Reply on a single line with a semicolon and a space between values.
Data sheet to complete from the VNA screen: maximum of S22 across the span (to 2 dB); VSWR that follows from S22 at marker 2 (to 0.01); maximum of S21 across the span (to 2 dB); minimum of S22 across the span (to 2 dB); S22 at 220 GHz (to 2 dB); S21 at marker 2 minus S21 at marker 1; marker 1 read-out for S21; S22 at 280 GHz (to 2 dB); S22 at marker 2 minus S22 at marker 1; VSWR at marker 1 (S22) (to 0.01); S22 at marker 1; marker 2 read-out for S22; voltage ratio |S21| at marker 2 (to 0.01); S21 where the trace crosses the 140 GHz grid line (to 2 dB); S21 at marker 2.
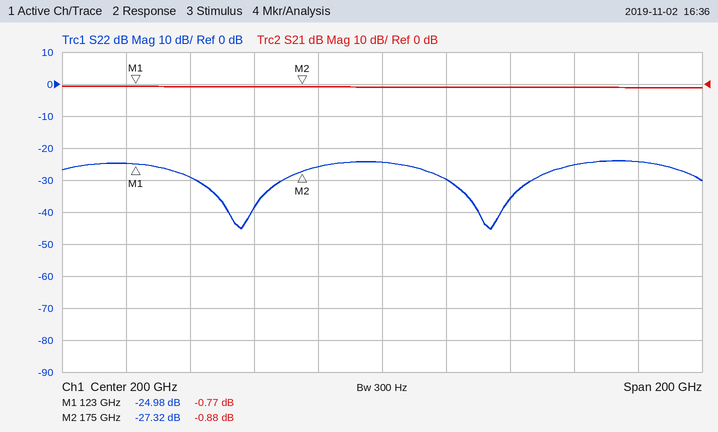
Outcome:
-24 dB; 1.09; 0 dB; -46 dB; -30 dB; -0.11 dB; -0.77 dB; -24 dB; -2.34 dB; 1.12; -24.98 dB; -27.32 dB; 0.90; 0 dB; -0.88 dB
